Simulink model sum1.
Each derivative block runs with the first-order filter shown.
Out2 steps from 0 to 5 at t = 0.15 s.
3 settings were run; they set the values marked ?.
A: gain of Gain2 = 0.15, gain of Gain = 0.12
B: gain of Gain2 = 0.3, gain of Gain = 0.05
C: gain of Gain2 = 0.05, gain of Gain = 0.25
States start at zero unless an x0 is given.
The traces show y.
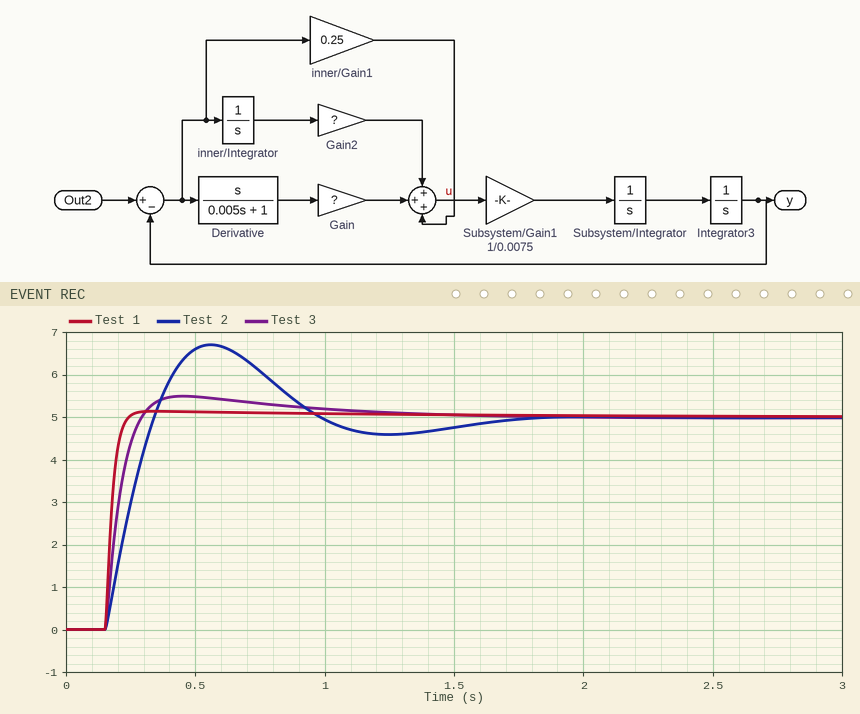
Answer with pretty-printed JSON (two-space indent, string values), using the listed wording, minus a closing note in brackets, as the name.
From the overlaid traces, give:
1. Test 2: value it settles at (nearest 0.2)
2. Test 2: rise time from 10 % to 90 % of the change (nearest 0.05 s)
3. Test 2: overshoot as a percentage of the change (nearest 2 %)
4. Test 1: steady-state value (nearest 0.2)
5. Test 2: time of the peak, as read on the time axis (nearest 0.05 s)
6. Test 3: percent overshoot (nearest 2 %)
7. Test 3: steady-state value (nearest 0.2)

{
  "Test 2: value it settles at": "5.0",
  "Test 2: rise time from 10 % to 90 % of the change": "0.15 s",
  "Test 2: overshoot as a percentage of the change": "34 %",
  "Test 1: steady-state value": "5.0",
  "Test 2: time of the peak, as read on the time axis": "0.55 s",
  "Test 3: percent overshoot": "10 %",
  "Test 3: steady-state value": "5.0"
}
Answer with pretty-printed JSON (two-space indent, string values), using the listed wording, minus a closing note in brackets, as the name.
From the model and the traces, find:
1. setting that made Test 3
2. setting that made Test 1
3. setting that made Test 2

{
  "setting that made Test 3": "A",
  "setting that made Test 1": "C",
  "setting that made Test 2": "B"
}
